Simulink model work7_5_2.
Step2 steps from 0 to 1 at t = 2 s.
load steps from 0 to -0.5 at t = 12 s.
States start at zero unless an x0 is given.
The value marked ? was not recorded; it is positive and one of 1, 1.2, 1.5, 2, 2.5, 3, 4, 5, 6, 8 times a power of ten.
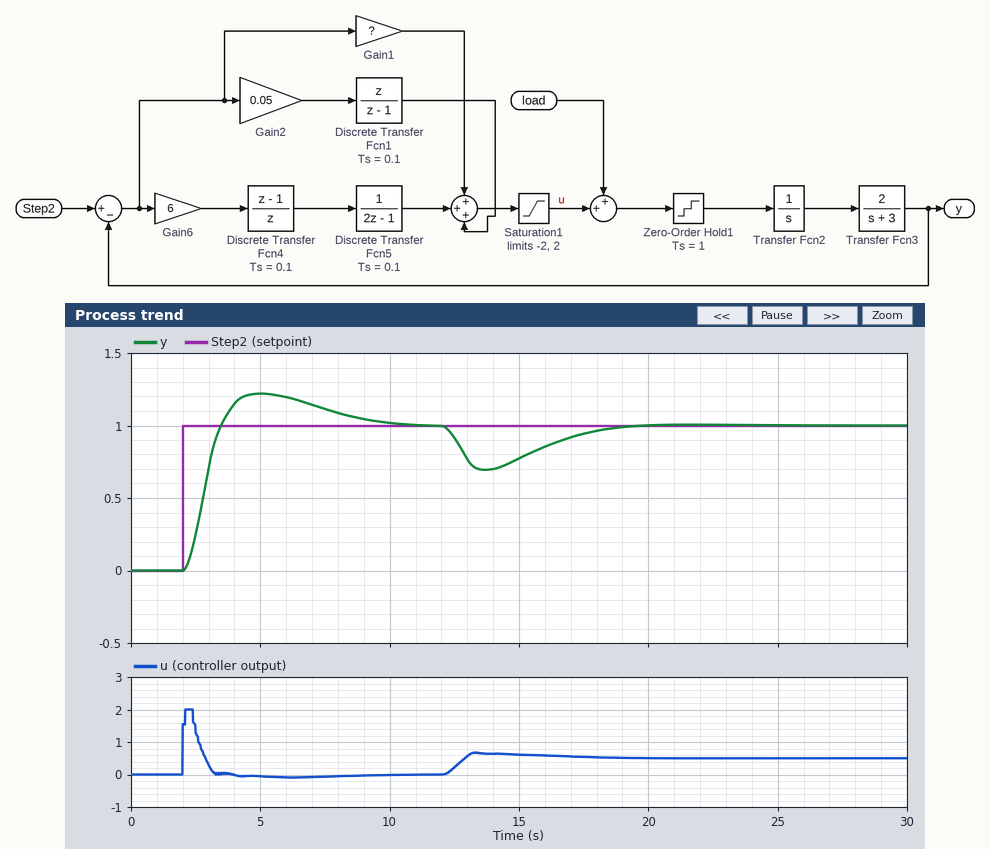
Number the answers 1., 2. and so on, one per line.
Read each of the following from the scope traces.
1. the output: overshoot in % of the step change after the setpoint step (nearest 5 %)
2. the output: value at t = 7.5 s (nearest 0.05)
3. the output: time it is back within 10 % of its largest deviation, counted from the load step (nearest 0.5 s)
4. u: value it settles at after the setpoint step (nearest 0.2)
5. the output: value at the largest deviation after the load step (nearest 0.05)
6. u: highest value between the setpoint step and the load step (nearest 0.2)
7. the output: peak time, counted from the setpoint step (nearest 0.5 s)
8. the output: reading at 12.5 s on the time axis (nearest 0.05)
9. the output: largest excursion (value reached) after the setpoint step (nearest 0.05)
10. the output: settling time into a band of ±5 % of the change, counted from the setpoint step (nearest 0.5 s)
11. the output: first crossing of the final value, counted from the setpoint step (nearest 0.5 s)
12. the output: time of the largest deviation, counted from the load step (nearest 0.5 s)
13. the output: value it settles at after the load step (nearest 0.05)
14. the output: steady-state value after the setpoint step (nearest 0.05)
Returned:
1. 20 %
2. 1.10
3. 6.0 s
4. 0.0
5. 0.70
6. 2.0
7. 3.0 s
8. 0.90
9. 1.20
10. 7.0 s
11. 1.5 s
12. 1.5 s
13. 1.00
14. 1.00
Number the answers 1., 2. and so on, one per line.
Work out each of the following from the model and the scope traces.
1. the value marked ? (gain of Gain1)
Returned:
1. 1.5
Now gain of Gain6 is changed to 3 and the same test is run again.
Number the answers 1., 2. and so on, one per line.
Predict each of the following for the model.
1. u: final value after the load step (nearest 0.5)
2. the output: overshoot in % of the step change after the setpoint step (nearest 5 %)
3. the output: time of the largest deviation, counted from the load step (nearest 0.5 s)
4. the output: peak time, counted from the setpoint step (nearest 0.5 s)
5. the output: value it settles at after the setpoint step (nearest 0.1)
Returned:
1. 0.5
2. 35 %
3. 2.0 s
4. 2.5 s
5. 1.0
